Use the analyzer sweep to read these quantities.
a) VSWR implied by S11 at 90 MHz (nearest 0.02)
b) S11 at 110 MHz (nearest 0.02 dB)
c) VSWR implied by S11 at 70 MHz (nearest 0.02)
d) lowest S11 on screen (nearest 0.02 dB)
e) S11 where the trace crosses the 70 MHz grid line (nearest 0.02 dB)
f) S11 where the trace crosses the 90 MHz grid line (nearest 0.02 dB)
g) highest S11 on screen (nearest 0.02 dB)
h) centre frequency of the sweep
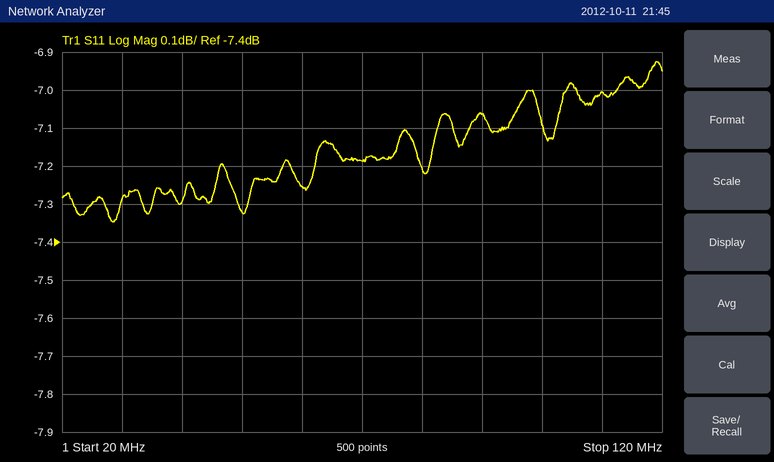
2.60
-7.00 dB
2.56
-7.34 dB
-7.18 dB
-7.06 dB
-6.92 dB
70 MHz
